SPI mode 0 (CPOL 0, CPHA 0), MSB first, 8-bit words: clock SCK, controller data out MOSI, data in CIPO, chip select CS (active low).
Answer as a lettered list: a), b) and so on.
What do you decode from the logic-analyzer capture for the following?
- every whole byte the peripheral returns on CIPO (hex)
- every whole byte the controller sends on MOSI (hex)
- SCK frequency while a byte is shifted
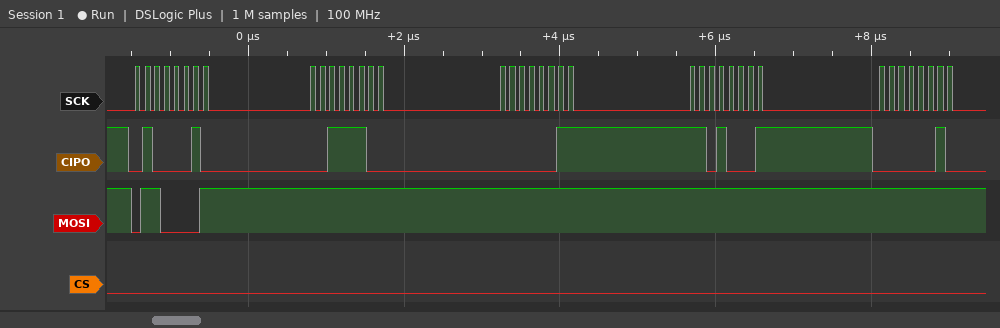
a) 0x42 0x3C 0x03 0xD1 0x02
b) 0x61 0xFF 0xFF 0xFF 0xFF
c) 8 MHz
